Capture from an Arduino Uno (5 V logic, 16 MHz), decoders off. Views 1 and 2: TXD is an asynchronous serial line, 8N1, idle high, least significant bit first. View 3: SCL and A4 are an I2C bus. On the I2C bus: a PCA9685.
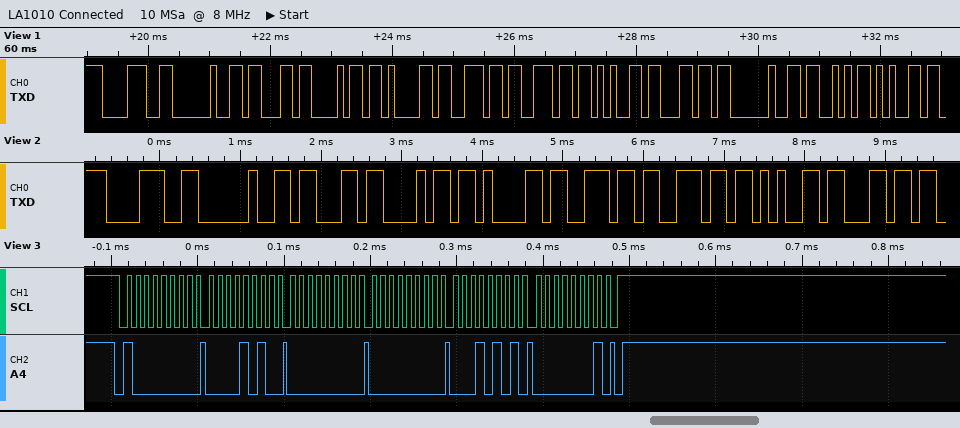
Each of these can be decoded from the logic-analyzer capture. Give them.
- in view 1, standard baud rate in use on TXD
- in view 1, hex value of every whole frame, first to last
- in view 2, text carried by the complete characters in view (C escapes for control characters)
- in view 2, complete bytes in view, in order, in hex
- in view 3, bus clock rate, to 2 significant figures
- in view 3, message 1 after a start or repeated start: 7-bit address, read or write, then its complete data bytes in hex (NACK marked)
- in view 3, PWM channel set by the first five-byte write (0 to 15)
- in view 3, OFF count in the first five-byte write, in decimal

9600 baud
38 20 63 68 61 6E 6E 65 6C 20 53 65
"8 channel"
0x38 0x20 0x63 0x68 0x61 0x6E 0x6E 0x65 0x6C
100 kHz
0x40 write: 0A 00 00 15 01
1
277
